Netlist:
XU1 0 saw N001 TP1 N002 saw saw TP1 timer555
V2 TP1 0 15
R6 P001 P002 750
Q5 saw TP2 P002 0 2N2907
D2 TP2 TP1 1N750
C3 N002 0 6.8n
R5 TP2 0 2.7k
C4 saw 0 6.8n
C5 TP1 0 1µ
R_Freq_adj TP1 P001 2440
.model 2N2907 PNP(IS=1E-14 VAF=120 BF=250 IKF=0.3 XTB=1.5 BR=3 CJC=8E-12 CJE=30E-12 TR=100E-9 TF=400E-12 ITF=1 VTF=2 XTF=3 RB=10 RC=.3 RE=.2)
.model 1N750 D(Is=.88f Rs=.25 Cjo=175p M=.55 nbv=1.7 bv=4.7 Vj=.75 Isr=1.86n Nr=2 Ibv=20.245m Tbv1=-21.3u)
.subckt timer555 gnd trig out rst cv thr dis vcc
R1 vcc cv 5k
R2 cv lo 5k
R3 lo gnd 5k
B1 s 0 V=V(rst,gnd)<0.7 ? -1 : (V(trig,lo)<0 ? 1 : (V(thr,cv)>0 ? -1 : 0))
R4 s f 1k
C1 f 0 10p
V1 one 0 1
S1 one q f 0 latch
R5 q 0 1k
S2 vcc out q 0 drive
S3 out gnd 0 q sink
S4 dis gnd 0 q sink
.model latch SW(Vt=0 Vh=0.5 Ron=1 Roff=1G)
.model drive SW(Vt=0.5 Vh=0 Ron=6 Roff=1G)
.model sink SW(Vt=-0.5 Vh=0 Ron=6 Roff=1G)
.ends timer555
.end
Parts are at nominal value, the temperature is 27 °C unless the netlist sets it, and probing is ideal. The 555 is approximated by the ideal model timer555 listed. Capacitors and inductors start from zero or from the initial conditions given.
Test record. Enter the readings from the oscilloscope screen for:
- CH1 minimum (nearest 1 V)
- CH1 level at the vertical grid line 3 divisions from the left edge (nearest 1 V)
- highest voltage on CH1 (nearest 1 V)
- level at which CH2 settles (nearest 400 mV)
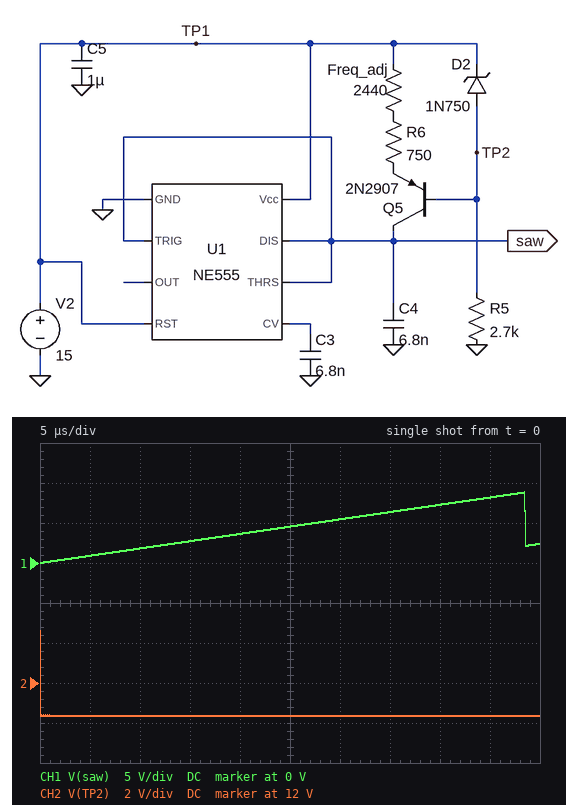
0 V
3 V
9 V
10.4 V
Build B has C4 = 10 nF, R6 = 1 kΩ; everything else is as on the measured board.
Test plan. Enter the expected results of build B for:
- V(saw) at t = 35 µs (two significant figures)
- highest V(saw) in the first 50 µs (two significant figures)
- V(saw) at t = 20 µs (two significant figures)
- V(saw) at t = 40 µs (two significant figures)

4.0 V
5.7 V
2.3 V
4.6 V
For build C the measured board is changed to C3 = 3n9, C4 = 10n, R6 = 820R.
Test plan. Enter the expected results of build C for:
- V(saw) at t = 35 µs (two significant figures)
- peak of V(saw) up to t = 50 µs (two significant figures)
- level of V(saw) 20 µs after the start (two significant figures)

4.2 V
6.1 V
2.4 V
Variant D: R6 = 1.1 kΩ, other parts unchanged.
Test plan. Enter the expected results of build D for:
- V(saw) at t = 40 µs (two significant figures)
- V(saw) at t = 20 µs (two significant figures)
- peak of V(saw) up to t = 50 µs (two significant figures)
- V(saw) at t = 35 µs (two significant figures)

6.6 V
3.3 V
8.2 V
5.7 V
